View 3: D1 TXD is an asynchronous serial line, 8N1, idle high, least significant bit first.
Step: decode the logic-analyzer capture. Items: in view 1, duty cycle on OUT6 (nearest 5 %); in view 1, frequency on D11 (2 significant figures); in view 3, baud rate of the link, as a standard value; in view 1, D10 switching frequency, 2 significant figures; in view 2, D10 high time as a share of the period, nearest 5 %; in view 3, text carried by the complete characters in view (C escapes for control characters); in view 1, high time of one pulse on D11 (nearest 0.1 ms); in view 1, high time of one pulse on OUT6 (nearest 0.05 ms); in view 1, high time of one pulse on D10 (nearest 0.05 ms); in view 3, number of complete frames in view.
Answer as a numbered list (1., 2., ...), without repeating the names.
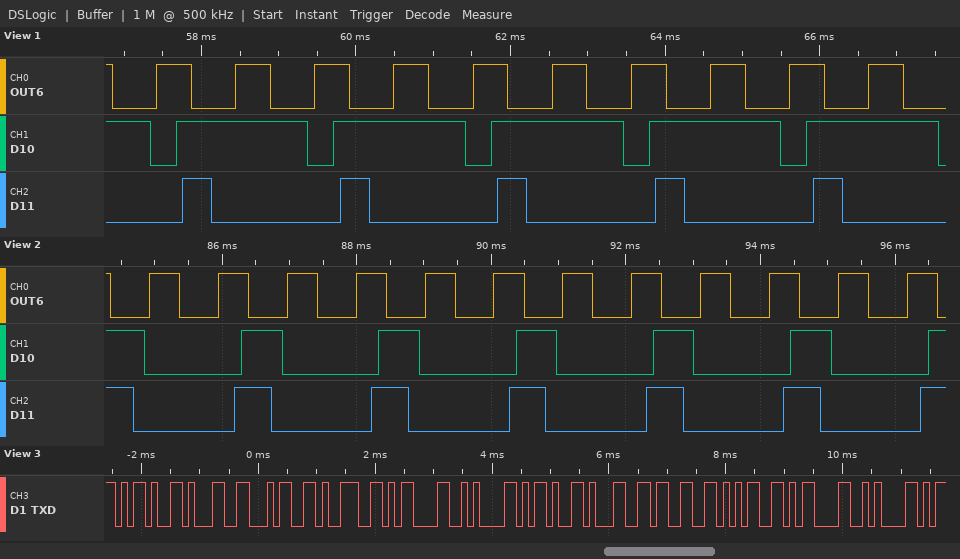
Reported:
1. 45 %
2. 490 Hz
3. 9600 baud
4. 490 Hz
5. 30 %
6. "-149\r\n-135\r\n"
7. 0.4 ms
8. 0.45 ms
9. 1.70 ms
10. 12
